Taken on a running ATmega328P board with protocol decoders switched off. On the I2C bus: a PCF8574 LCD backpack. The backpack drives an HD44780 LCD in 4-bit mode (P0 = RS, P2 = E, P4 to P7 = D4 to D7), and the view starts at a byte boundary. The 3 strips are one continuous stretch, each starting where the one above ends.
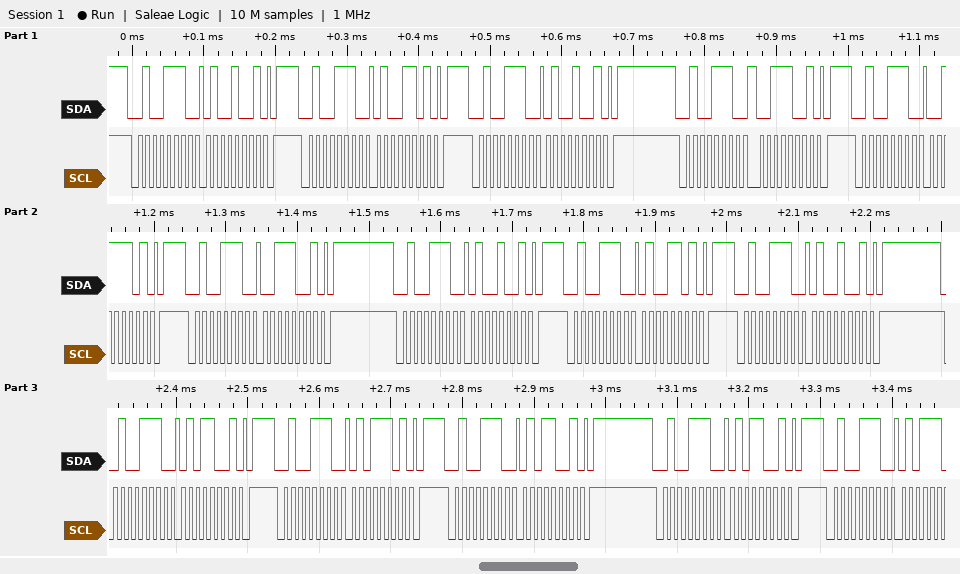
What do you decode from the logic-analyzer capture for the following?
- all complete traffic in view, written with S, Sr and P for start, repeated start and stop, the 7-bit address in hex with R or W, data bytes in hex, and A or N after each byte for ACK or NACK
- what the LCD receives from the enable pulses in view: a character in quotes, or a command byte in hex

S 27W A 49 A P S 27W A 4D A P S 27W A 49 A P S 27W A 39 A P S 27W A 3D A P S 27W A 39 A P S 27W A 49 A P S 27W A 4D A P S 27W A 49 A P S 27W A 59 A P S 27W A 5D A P S 27W A 59 A P S 27W A 59 A P S 27W A
'C' 'E'
